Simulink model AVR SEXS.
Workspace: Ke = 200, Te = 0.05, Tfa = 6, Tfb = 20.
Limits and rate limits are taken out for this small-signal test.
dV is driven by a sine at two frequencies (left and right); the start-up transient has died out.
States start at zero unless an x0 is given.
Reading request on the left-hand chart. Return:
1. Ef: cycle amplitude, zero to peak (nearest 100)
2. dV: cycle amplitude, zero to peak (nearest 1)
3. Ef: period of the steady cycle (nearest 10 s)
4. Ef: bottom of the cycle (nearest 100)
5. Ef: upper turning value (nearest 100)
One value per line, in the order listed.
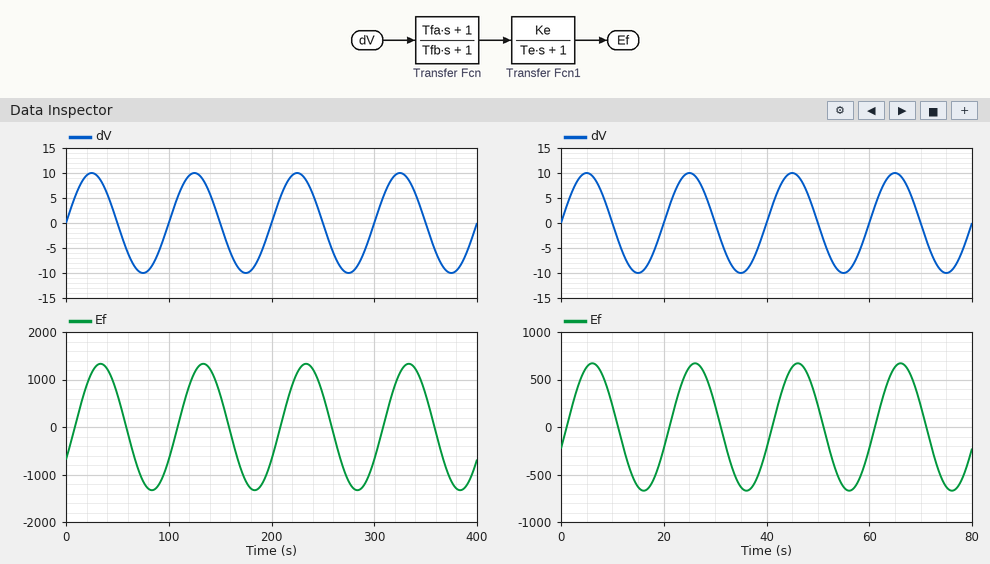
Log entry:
1300
10
100 s
-1300
1300
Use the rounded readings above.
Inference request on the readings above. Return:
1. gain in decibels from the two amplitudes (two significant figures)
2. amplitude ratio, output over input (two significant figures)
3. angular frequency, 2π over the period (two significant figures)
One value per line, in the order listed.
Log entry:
42 dB
130
0.063 rad/s
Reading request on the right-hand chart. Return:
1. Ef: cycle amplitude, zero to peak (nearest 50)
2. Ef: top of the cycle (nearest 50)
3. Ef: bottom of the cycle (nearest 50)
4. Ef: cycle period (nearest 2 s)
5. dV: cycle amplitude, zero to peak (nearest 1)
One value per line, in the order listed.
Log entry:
650
650
-650
20 s
10
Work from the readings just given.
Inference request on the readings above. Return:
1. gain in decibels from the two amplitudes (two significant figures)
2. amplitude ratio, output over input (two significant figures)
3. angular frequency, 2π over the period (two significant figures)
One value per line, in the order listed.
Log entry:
36 dB
65
0.31 rad/s
